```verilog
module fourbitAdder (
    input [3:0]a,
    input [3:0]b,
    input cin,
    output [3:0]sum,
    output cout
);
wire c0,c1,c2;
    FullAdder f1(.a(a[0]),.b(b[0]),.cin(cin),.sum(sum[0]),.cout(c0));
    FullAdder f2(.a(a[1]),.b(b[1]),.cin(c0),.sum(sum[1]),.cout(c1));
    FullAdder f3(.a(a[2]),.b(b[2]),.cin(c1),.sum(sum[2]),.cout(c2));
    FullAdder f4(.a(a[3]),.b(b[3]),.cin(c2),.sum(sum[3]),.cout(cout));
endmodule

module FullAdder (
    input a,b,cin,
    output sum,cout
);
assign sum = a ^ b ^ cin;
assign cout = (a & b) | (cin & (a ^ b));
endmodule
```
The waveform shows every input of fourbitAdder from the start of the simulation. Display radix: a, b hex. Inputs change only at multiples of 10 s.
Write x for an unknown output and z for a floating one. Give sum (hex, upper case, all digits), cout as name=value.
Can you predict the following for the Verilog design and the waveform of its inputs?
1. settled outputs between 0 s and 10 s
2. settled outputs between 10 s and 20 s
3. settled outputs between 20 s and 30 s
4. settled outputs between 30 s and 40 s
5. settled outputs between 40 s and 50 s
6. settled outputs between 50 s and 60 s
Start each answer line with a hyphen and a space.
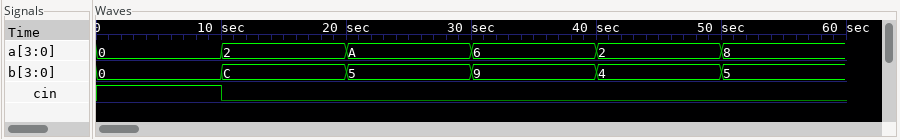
- sum=1, cout=0
- sum=E, cout=0
- sum=F, cout=0
- sum=F, cout=0
- sum=6, cout=0
- sum=D, cout=0
